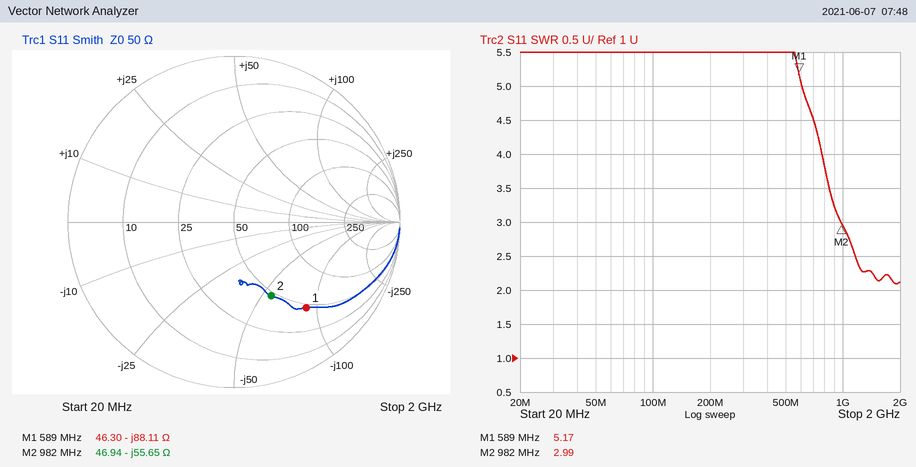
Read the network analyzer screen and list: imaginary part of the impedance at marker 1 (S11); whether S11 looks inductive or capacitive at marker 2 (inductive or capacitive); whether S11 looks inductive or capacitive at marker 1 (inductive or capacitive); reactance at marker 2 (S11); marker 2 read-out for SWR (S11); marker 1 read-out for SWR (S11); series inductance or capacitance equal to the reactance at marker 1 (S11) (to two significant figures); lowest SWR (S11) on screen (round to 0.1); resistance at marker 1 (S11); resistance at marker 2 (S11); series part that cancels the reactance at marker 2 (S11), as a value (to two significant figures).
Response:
-88.11 Ω
capacitive
capacitive
-55.65 Ω
2.99
5.17
3.1 pF
2.1
46.30 Ω
46.94 Ω
9.0 nH
